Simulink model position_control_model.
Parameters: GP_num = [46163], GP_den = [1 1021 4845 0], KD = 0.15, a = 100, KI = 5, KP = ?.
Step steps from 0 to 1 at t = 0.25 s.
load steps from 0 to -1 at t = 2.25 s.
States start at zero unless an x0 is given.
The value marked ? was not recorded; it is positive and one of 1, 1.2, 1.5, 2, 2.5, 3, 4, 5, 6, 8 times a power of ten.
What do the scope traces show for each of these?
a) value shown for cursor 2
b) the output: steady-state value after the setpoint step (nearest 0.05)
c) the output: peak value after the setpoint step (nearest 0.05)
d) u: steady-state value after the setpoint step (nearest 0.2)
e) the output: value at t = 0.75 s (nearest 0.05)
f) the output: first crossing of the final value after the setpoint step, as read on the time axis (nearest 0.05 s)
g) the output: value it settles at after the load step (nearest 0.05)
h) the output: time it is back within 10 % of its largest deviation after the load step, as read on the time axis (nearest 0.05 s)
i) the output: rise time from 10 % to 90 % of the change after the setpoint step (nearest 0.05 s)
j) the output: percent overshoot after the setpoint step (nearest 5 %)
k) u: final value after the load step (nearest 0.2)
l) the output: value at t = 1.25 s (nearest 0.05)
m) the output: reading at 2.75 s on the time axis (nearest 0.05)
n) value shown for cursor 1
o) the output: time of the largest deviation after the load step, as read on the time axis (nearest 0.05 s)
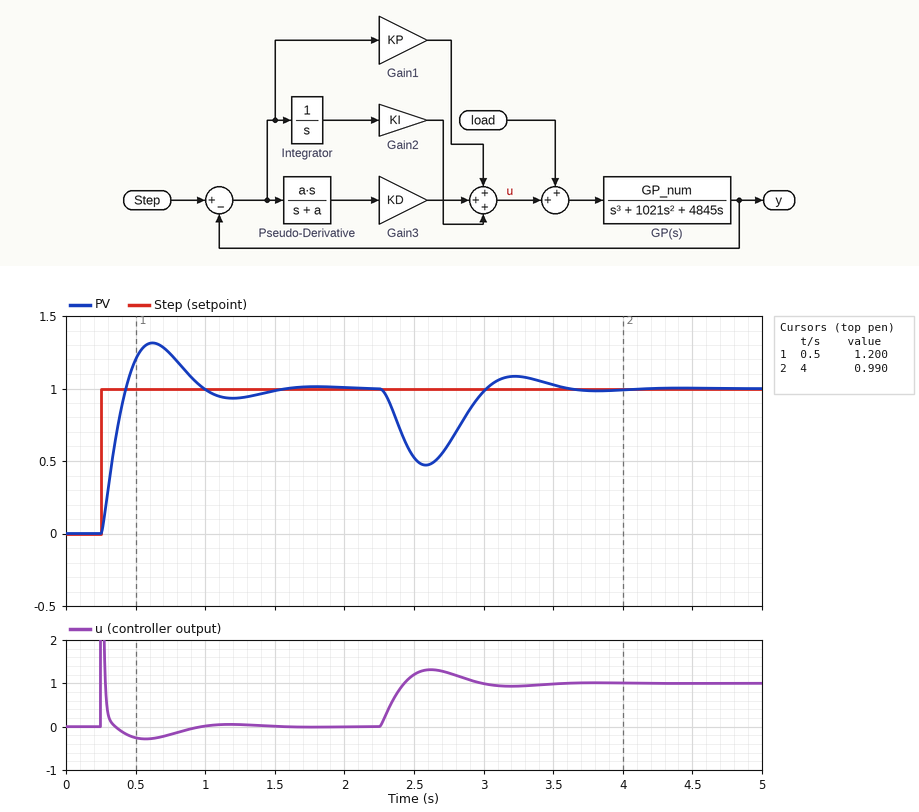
0.990
1.00
1.30
0.0
1.25
0.45 s
1.00
3.40 s
0.15 s
30 %
1.0
0.95
0.60
1.200
2.60 s
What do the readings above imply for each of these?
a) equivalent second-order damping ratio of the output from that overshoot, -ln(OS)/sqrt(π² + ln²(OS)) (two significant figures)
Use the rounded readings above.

0.36
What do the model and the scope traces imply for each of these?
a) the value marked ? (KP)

1.5
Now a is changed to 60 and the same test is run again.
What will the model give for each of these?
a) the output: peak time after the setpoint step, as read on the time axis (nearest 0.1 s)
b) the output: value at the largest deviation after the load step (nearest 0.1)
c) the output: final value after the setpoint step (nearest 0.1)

0.6 s
0.5
1.0
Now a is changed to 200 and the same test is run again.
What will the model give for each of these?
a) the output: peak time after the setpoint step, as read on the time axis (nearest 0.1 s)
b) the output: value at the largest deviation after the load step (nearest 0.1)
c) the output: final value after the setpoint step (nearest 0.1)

0.6 s
0.5
1.0
